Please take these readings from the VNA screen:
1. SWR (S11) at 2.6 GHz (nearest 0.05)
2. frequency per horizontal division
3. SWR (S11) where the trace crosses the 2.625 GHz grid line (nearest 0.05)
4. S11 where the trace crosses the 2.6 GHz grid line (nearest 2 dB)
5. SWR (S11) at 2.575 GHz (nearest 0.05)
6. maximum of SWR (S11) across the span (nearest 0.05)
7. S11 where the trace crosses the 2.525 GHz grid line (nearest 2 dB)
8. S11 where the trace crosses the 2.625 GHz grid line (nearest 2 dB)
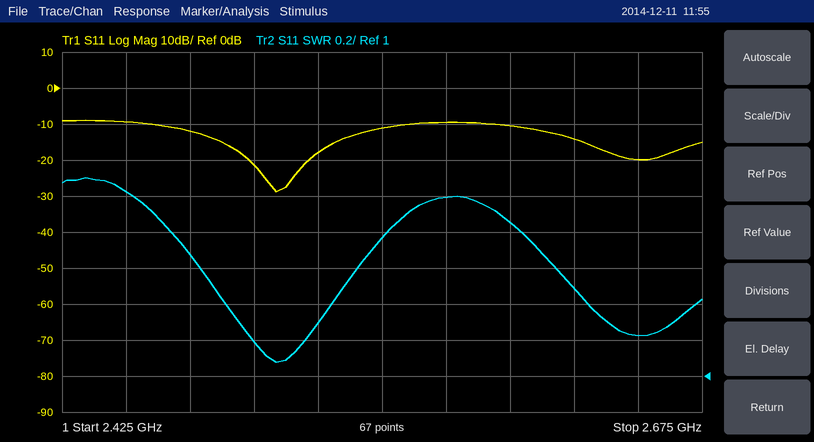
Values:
1.85
25 MHz
1.50
-10 dB
2.00
2.10
-18 dB
-14 dB
